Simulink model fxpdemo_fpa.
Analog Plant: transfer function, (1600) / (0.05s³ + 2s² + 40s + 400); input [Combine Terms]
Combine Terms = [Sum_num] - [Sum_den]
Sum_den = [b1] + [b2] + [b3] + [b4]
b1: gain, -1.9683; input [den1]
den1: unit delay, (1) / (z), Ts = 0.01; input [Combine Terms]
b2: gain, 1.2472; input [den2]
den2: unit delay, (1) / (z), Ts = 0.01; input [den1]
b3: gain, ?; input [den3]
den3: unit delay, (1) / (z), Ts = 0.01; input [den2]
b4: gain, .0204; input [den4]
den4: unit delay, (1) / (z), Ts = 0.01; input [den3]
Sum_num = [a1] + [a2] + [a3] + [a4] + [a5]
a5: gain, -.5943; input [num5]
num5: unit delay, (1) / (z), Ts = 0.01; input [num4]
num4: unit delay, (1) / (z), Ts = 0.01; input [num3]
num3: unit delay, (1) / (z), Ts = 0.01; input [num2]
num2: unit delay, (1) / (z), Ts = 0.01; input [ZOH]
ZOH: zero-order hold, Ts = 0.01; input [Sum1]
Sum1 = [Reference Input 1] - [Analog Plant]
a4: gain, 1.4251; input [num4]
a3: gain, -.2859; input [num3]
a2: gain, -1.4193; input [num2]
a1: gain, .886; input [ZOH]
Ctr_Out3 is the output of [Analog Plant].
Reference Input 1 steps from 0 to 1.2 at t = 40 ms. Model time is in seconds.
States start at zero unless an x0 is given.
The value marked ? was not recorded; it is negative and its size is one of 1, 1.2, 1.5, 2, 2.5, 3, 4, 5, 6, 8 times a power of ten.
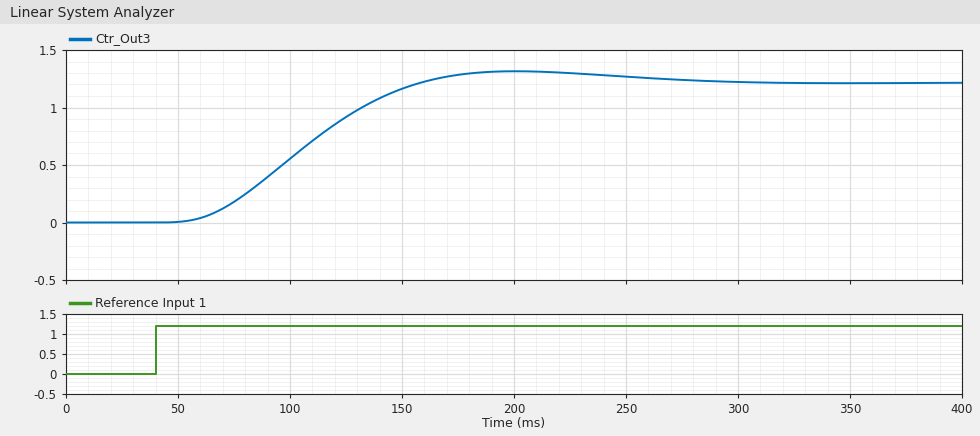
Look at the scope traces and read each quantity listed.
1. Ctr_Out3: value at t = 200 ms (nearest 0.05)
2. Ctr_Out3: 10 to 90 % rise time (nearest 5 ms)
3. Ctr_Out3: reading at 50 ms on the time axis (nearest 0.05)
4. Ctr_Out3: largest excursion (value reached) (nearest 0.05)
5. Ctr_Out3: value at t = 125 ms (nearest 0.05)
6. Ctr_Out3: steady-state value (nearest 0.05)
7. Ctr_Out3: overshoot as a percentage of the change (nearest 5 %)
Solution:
1.30
70 ms
0.00
1.30
0.90
1.20
10 %
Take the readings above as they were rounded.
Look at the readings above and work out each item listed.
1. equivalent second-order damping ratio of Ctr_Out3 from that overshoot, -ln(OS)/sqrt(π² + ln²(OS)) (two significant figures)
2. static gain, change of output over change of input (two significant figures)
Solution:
0.59
1.0
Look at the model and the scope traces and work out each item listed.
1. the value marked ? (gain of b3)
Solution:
-0.3
